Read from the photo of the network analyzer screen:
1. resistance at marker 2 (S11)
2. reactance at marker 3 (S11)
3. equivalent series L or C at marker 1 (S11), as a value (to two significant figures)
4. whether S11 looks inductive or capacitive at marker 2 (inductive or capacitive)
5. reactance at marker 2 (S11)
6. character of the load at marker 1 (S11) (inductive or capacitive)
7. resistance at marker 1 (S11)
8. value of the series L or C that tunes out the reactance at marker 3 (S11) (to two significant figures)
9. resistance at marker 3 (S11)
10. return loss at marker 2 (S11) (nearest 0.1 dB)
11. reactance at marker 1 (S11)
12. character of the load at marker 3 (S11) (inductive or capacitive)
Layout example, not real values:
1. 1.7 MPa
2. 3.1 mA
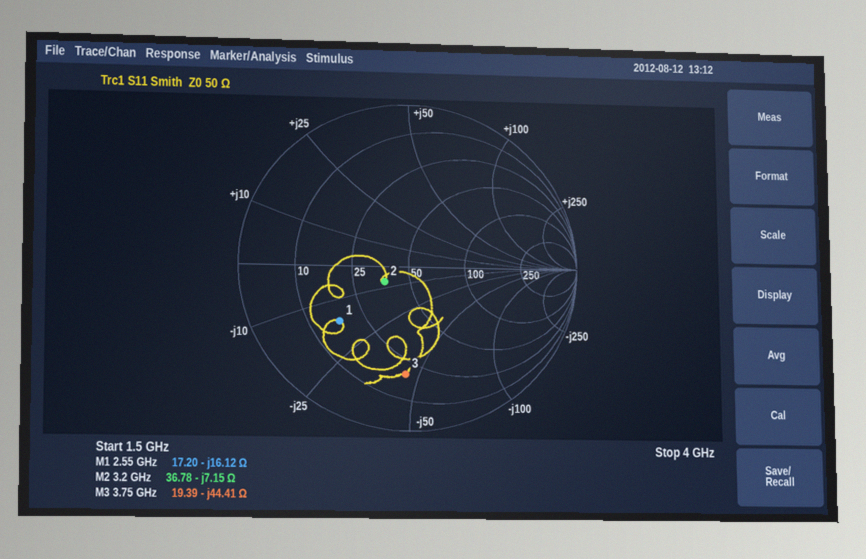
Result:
1. 36.78 Ω
2. -44.41 Ω
3. 3.9 pF
4. capacitive
5. -7.15 Ω
6. capacitive
7. 17.20 Ω
8. 1.9 nH
9. 19.39 Ω
10. 15.3 dB
11. -16.12 Ω
12. capacitive
